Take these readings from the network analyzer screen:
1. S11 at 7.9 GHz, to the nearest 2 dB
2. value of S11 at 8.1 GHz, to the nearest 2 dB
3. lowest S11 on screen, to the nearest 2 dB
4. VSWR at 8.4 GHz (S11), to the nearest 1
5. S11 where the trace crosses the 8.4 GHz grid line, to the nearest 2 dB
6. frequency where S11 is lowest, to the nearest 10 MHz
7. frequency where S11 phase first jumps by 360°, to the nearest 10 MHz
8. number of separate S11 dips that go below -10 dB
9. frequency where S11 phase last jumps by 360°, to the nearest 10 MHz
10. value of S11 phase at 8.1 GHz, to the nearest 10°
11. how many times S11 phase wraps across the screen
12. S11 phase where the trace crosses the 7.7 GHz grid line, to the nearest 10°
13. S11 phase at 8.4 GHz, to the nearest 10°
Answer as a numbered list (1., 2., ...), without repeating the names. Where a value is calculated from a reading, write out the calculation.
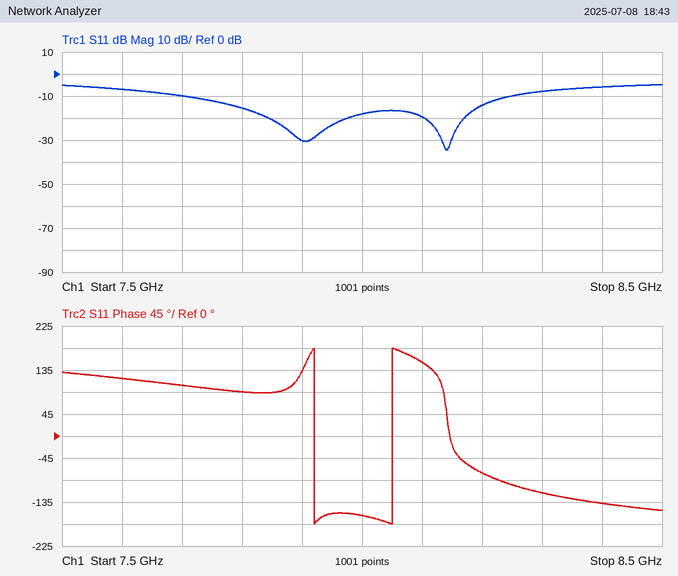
1. -30 dB
2. -20 dB
3. -34 dB
4. |Γ| = 10^(-6/20) = 0.5012; VSWR = (1 + 0.5012)/(1 − 0.5012) ≈ 3
5. -6 dB
6. 8.14 GHz
7. 7.92 GHz
8. 2
9. 8.05 GHz
10. 150°
11. 2
12. 100°
13. -140°
